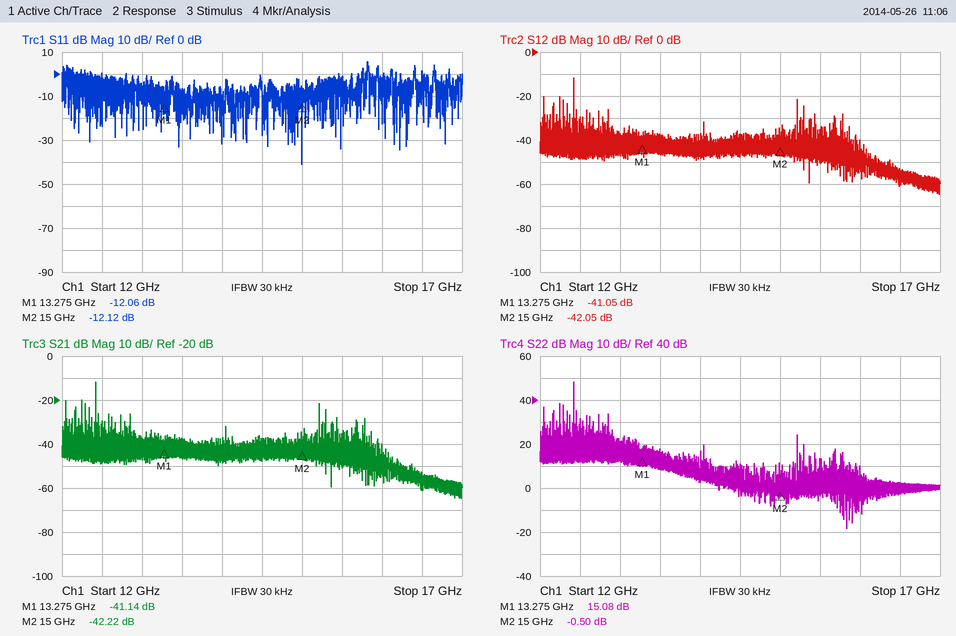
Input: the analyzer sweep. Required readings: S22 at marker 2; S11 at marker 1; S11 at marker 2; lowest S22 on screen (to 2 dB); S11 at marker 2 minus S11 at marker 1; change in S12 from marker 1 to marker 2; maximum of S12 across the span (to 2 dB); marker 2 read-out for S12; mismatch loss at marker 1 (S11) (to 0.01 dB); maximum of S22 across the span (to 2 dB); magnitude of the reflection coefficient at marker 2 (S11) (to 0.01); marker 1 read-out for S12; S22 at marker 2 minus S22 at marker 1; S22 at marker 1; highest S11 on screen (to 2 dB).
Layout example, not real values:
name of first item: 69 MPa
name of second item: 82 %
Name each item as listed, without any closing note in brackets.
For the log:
S22 at marker 2: -0.50 dB
S11 at marker 1: -12.06 dB
S11 at marker 2: -12.12 dB
lowest S22 on screen: -18 dB
S11 at marker 2 minus S11 at marker 1: -0.06 dB
change in S12 from marker 1 to marker 2: -1.00 dB
maximum of S12 across the span: -12 dB
marker 2 read-out for S12: -42.05 dB
mismatch loss at marker 1 (S11): 0.28 dB
maximum of S22 across the span: 48 dB
magnitude of the reflection coefficient at marker 2 (S11): 0.25
marker 1 read-out for S12: -41.05 dB
S22 at marker 2 minus S22 at marker 1: -15.58 dB
S22 at marker 1: 15.08 dB
highest S11 on screen: 6 dB
